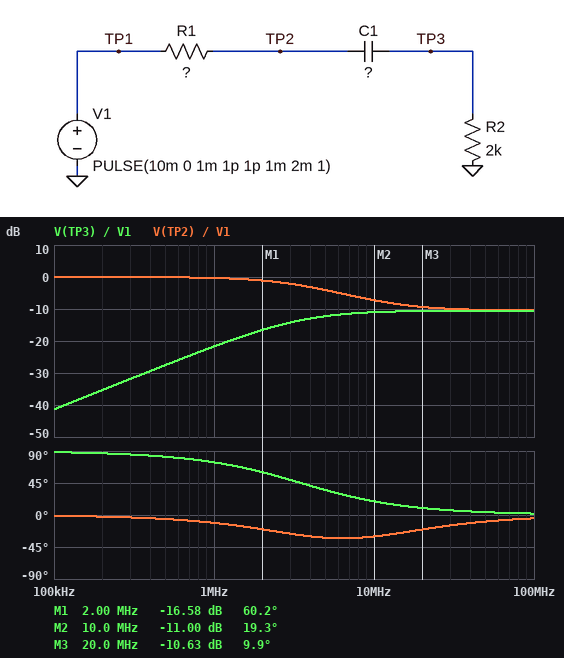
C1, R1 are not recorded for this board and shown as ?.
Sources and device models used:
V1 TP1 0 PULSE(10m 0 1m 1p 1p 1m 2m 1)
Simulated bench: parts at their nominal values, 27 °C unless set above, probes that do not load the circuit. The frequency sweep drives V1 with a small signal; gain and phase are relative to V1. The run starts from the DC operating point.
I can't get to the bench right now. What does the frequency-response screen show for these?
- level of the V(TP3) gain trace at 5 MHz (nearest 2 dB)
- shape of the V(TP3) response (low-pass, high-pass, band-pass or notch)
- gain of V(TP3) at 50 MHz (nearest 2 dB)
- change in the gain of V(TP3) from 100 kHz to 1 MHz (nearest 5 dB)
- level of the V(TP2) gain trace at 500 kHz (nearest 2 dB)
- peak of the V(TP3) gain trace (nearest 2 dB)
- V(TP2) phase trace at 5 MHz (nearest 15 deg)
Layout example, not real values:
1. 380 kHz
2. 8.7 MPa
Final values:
1. -12 dB
2. high-pass
3. -10 dB
4. 20 dB
5. 0 dB
6. -10 dB
7. -30 deg
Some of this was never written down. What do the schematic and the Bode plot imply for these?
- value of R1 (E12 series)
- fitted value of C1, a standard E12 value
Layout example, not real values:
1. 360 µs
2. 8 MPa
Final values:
1. 4.7 kΩ
2. 6.8 pF
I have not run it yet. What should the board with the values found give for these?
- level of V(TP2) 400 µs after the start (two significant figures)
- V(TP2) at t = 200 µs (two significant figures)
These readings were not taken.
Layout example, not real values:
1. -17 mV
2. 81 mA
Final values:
1. 10 mV
2. 10 mV
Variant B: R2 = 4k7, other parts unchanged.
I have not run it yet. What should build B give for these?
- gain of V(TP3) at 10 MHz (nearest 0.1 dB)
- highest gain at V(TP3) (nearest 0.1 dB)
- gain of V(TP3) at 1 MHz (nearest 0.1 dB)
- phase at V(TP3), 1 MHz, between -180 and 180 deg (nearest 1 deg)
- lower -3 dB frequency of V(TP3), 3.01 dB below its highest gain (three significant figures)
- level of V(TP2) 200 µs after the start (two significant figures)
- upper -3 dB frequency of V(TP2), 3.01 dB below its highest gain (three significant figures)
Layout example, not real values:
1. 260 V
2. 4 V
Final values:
1. -6.3 dB
2. -6.0 dB
3. -14.6 dB
4. 68 deg
5. 2.49 MHz
6. 10 mV
7. 3.52 MHz
